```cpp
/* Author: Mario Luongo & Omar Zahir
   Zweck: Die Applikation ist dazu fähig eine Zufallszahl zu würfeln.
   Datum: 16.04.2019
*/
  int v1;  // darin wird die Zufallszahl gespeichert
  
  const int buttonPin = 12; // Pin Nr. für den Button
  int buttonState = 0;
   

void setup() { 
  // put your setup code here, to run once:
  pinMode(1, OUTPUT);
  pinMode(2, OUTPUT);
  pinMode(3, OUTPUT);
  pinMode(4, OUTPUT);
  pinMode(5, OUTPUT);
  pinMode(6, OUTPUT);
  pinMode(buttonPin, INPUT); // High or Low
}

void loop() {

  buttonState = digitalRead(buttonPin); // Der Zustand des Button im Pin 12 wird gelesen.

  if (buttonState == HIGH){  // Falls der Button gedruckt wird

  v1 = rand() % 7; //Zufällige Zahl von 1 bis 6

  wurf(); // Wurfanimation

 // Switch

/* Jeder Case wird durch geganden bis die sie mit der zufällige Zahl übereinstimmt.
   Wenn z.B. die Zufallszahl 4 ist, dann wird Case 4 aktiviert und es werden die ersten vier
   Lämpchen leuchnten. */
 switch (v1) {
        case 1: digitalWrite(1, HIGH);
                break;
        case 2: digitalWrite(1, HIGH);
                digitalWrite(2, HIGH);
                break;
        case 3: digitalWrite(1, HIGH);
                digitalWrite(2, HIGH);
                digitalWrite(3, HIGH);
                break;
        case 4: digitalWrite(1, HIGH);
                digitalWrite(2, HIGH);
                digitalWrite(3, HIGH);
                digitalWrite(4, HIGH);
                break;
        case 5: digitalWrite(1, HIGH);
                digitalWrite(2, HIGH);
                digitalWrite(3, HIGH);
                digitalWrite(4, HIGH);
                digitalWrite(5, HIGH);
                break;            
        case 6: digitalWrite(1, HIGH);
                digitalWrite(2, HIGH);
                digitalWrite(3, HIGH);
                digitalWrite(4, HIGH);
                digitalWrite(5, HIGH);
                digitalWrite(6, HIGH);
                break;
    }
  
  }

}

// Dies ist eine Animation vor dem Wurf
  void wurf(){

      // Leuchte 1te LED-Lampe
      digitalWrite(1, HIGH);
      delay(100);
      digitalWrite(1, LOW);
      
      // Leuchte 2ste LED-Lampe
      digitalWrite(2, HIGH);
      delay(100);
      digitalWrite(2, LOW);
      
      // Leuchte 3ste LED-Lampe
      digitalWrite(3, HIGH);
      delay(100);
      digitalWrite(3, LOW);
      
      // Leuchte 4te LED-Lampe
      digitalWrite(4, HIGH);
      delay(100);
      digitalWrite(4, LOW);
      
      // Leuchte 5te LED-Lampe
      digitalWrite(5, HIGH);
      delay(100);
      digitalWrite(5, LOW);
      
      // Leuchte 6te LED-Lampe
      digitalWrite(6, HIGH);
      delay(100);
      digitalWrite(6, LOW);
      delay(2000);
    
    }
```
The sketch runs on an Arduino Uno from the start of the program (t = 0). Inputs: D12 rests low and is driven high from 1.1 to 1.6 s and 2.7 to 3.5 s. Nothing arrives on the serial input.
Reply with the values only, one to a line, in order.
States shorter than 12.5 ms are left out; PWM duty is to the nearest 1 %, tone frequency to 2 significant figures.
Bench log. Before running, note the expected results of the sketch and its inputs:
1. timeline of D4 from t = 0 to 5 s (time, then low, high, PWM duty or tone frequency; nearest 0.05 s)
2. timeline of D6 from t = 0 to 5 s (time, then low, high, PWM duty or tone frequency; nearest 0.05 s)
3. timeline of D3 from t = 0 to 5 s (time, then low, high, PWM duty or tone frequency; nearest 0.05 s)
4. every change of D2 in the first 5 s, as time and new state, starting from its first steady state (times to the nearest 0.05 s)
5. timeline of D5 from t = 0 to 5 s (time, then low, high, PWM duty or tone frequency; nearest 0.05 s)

0 s low; 1.4 s high; 1.5 s low
0 s low; 1.6 s high; 1.7 s low
0 s low; 1.3 s high; 1.4 s low
0 s low; 1.2 s high; 1.3 s low
0 s low; 1.5 s high; 1.6 s low
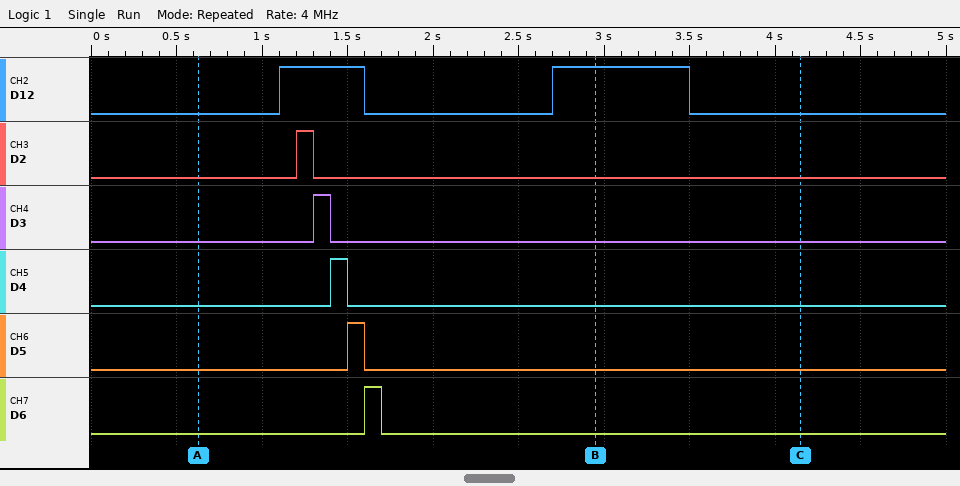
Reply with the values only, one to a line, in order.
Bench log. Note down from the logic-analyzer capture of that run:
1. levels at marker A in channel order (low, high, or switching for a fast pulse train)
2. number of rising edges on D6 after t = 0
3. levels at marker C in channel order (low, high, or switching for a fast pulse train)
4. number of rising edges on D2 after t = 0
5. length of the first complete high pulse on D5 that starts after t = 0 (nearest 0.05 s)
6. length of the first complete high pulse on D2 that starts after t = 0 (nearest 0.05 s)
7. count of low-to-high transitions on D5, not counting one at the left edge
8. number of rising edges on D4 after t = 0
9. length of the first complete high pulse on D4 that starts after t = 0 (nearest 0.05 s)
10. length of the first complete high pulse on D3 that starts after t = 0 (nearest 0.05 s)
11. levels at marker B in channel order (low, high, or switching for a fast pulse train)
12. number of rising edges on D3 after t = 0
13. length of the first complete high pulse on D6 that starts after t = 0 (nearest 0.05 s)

D12 low, D2 low, D3 low, D4 low, D5 low, D6 low
1
D12 low, D2 low, D3 low, D4 low, D5 low, D6 low
1
0.10 s
0.10 s
1
1
0.10 s
0.10 s
D12 high, D2 low, D3 low, D4 low, D5 low, D6 low
1
0.10 s
